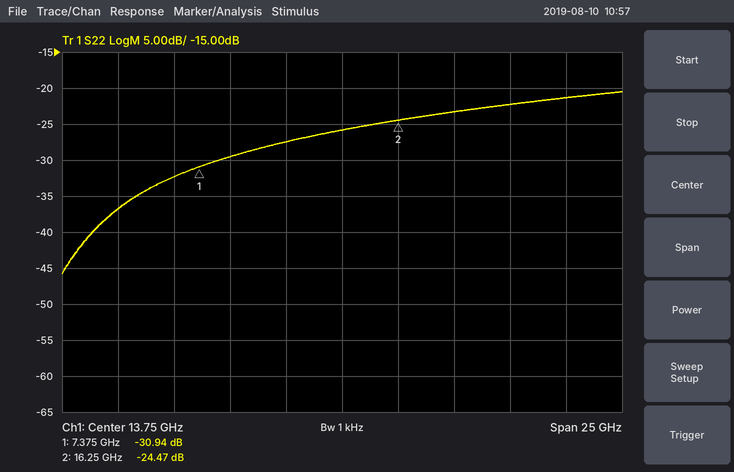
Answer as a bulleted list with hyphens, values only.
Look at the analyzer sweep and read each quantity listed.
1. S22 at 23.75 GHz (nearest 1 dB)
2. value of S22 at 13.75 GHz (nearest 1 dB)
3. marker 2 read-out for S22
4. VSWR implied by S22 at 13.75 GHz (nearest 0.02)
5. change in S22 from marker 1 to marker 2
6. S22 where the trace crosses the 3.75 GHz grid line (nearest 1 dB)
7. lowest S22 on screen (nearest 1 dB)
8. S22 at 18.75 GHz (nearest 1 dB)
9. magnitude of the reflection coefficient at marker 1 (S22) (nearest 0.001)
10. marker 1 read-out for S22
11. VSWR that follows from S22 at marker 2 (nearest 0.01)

- -21 dB
- -26 dB
- -24.47 dB
- 1.10
- 6.47 dB
- -37 dB
- -46 dB
- -23 dB
- 0.028
- -30.94 dB
- 1.13
